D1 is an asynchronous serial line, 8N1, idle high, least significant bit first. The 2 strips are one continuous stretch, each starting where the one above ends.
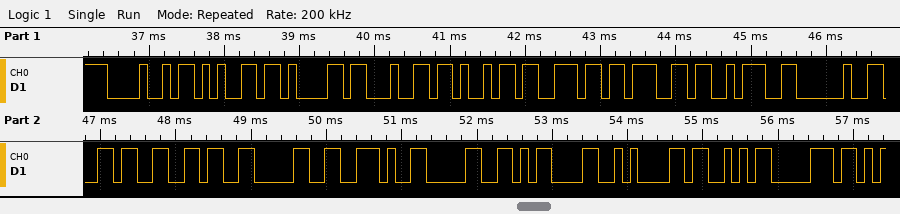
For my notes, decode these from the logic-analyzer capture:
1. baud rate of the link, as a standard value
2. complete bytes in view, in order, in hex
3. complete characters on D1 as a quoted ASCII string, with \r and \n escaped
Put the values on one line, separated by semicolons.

9600 baud; 48 65 61 64 69 6E 67 3A 20 36 36 30 2E 30 0D 0A 53 70; "Heading: 660.0\r\nSp"
